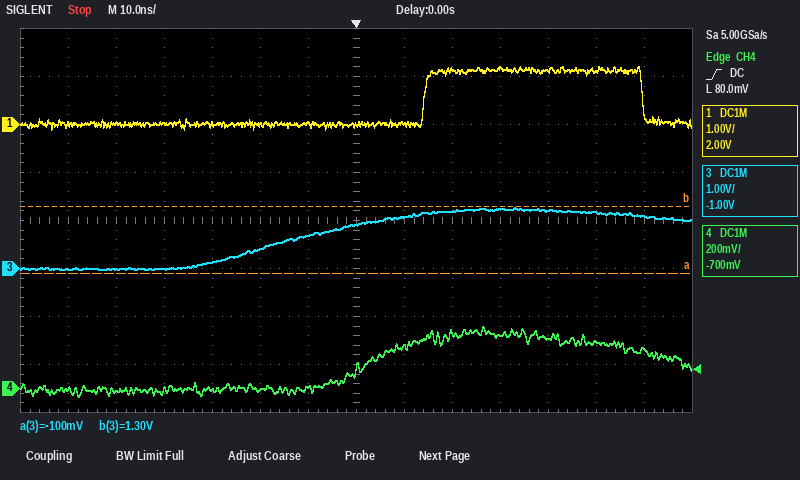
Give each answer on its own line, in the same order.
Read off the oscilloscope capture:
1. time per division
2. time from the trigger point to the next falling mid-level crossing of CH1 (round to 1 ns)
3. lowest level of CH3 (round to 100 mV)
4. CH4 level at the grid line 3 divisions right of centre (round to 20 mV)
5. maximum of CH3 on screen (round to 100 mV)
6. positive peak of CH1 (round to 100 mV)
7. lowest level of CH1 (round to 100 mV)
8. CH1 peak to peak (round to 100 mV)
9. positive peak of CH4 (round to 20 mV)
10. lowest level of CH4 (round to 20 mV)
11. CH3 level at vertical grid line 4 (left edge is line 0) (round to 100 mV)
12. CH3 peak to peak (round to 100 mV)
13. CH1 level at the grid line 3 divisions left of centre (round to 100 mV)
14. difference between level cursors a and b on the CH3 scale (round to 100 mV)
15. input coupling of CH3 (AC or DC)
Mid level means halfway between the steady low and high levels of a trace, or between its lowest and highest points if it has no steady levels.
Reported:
10 ns
60 ns
0.0 V
220 mV
1.3 V
1.2 V
-100 mV
1.3 V
260 mV
-40 mV
100 mV
1.3 V
0.0 V
1.4 V
DC
